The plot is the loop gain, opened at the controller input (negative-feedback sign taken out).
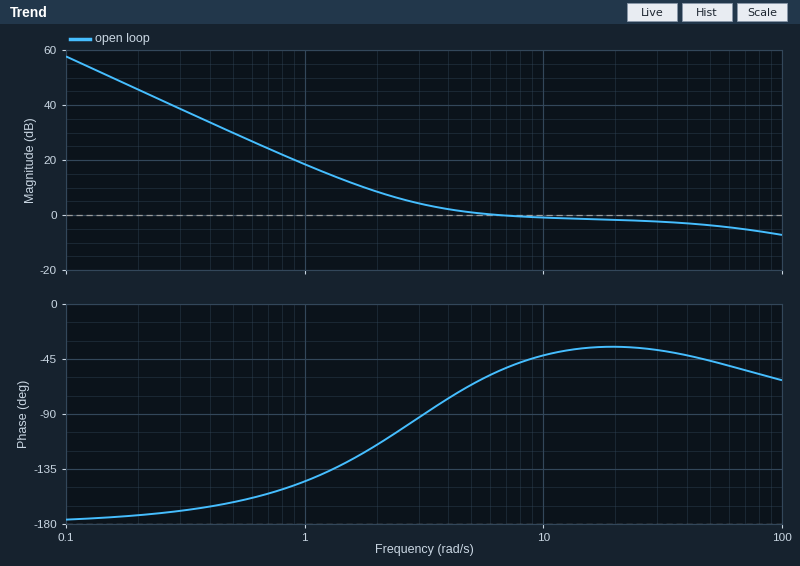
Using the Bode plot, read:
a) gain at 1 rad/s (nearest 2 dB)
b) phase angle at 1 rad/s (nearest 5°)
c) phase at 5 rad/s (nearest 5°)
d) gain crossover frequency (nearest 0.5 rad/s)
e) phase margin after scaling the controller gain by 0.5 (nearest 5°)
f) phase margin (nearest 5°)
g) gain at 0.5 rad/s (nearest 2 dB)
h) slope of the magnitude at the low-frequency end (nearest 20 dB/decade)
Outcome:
18 dB
-145°
-65°
6.5 rad/s
75°
125°
30 dB
-40 dB/decade
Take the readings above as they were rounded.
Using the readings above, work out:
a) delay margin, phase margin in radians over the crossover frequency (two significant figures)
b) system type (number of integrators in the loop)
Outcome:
0.34 s
2
